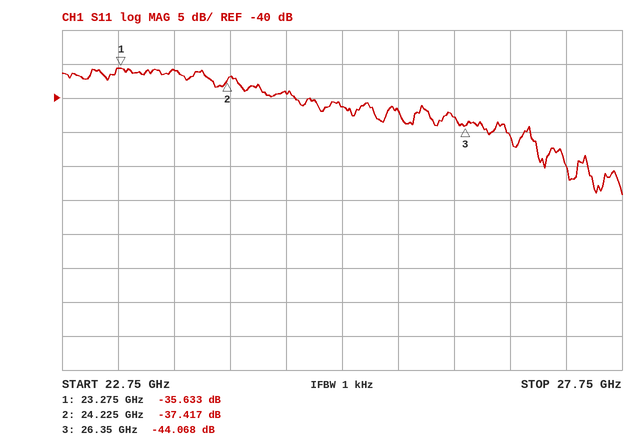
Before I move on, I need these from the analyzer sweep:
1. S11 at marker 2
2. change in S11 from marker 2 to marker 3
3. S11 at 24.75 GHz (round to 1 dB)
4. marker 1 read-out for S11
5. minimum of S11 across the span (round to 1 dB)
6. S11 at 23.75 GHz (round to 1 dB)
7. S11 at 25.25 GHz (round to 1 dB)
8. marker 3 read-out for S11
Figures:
-37.417 dB
-6.651 dB
-39 dB
-35.633 dB
-54 dB
-36 dB
-41 dB
-44.068 dB
